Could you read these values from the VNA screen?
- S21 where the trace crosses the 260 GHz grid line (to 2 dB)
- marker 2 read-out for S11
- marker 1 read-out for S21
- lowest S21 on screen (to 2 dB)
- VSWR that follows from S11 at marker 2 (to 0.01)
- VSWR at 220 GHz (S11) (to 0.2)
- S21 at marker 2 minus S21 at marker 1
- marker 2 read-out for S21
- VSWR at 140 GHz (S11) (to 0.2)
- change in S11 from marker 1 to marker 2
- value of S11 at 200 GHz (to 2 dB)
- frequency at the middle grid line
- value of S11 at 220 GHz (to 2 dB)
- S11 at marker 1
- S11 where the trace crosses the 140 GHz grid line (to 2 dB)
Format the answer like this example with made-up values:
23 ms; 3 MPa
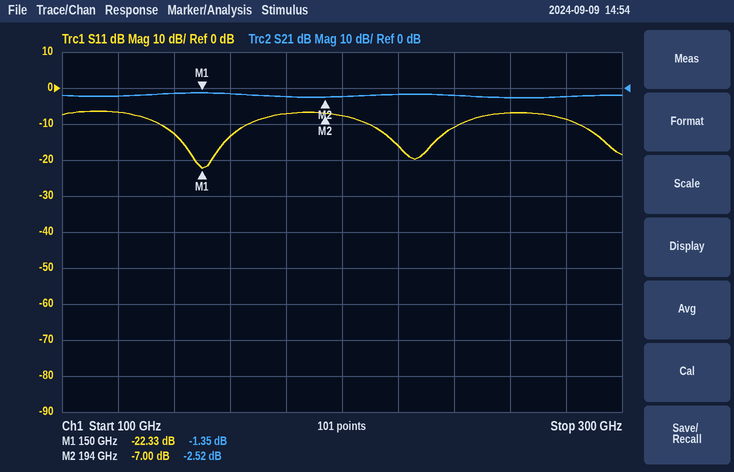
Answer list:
-2 dB; -7.00 dB; -1.35 dB; -2 dB; 2.61; 1.4; -1.17 dB; -2.52 dB; 1.6; 15.33 dB; -8 dB; 200 GHz; -16 dB; -22.33 dB; -12 dB
